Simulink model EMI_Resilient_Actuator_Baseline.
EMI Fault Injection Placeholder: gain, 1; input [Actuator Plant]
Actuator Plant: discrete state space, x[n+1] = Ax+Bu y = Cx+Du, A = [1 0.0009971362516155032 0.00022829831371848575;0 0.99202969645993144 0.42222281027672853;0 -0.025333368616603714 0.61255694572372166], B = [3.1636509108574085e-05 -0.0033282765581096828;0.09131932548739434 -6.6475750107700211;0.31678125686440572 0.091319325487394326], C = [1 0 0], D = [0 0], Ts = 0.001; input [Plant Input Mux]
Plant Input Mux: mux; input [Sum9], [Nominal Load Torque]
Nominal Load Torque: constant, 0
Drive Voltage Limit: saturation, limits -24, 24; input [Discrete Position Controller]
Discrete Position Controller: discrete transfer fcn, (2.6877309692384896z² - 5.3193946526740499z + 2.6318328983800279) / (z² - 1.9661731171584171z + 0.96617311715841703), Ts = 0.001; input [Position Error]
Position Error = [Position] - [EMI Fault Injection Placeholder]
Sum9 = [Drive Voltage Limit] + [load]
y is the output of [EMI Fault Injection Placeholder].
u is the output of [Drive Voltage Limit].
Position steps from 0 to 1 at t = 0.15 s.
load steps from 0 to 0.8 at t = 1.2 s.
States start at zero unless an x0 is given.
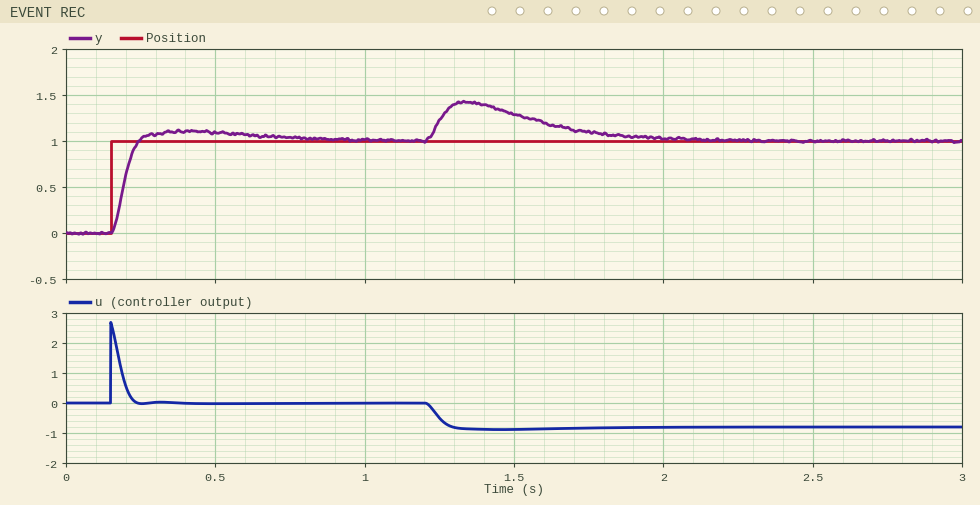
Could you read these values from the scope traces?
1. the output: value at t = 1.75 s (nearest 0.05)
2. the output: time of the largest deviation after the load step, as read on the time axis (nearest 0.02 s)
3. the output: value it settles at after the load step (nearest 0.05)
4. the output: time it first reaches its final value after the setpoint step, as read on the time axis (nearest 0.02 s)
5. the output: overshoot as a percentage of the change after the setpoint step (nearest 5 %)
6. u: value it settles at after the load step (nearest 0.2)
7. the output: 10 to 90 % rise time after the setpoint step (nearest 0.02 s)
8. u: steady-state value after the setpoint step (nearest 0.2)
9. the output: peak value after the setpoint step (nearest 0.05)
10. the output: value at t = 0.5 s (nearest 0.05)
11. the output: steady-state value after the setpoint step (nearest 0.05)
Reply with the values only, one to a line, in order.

1.10
1.34 s
1.00
0.24 s
10 %
-0.8
0.06 s
0.0
1.10
1.10
1.00
